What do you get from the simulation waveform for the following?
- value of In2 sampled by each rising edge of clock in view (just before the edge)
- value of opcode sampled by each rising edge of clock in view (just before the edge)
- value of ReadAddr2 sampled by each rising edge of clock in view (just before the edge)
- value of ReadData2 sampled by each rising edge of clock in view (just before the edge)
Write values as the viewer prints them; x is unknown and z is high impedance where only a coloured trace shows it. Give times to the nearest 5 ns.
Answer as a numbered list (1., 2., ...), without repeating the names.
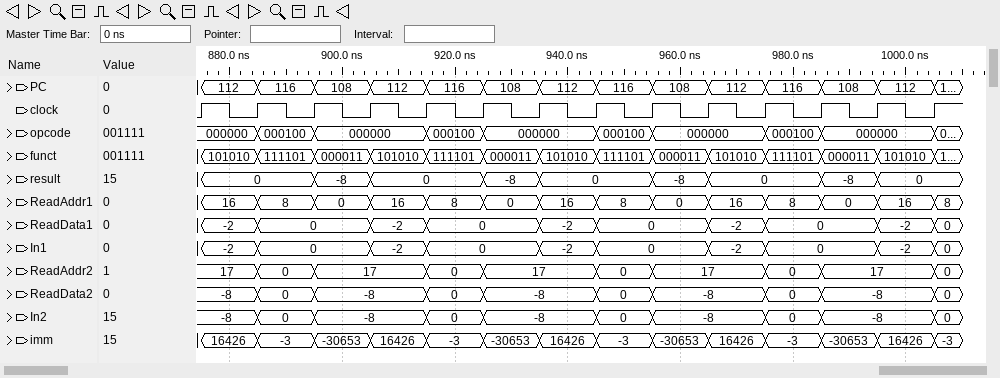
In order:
1. -8, -8, 0, -8, -8, 0, -8, -8, 0, -8, -8, 0, -8, -8
2. 000000, 000000, 000100, 000000, 000000, 000100, 000000, 000000, 000100, 000000, 000000, 000100, 000000, 000000
3. 17, 17, 0, 17, 17, 0, 17, 17, 0, 17, 17, 0, 17, 17
4. -8, -8, 0, -8, -8, 0, -8, -8, 0, -8, -8, 0, -8, -8
